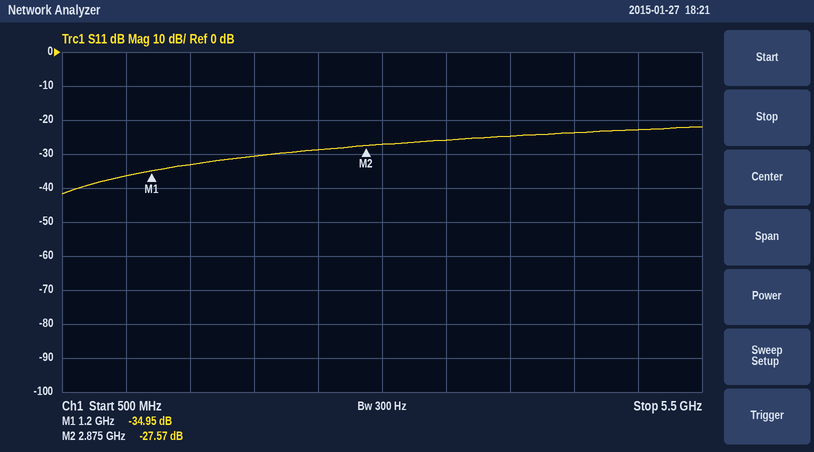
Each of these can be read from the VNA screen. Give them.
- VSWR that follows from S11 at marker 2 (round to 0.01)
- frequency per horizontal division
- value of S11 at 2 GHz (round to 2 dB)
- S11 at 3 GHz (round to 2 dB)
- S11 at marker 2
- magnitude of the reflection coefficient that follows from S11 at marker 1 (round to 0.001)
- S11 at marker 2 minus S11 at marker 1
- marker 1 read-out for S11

1.09
500 MHz
-30 dB
-28 dB
-27.57 dB
0.018
7.38 dB
-34.95 dB
